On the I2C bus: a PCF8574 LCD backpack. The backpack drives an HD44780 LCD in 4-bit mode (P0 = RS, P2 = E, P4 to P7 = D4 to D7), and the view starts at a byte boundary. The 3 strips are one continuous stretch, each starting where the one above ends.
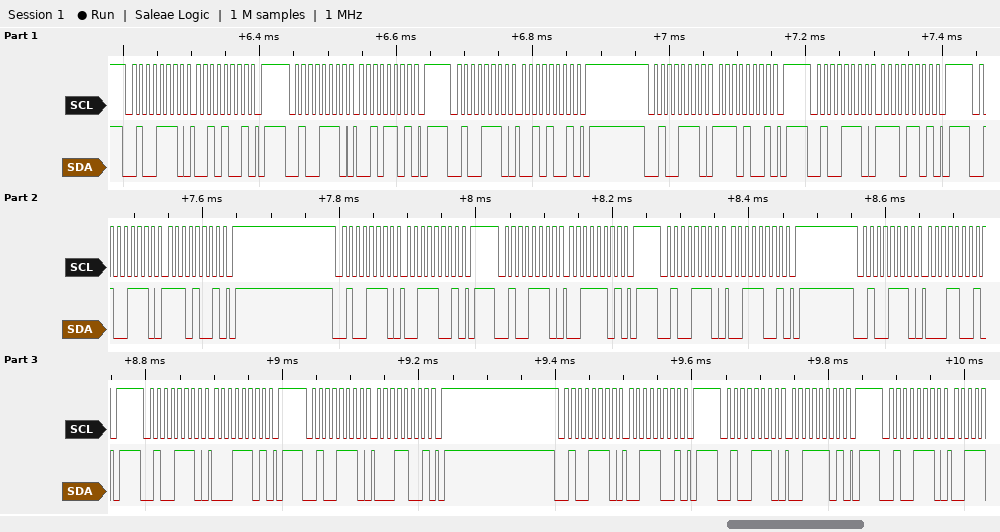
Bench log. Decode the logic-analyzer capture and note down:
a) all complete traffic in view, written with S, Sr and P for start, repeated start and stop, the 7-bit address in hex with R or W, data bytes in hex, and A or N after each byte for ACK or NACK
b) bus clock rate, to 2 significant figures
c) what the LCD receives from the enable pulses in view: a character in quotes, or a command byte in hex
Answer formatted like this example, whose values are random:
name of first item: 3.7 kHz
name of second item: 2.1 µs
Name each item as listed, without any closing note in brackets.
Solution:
all complete traffic in view, written with S, Sr and P for start, repeated start and stop, the 7-bit address in hex with R or W, data bytes in hex, and A or N after each byte for ACK or NACK: S 27W A 29 A P S 27W A 2D A P S 27W A 29 A P S 27W A E9 A P S 27W A ED A P S 27W A E9 A P S 27W A 39 A P S 27W A 3D A P S 27W A 39 A P S 27W A 19 A P S 27W A 1D A P S 27W A 19 A P S 27W A 39 A P S 27W A 3D A P S 27W A
bus clock rate, to 2 significant figures: 100 kHz
what the LCD receives from the enable pulses in view: a character in quotes, or a command byte in hex: '.' '1'
